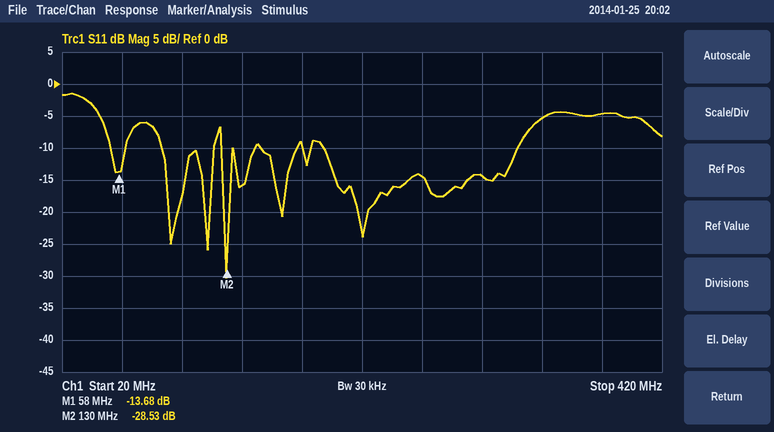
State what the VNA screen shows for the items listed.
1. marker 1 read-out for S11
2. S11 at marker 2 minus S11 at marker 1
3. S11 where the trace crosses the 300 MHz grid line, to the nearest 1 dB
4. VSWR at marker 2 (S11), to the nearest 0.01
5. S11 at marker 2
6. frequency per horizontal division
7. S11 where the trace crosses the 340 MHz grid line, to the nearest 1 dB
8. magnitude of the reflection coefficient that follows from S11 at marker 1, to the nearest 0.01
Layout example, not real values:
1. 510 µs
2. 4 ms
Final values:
1. -13.68 dB
2. -14.85 dB
3. -14 dB
4. 1.08
5. -28.53 dB
6. 40 MHz
7. -5 dB
8. 0.21
